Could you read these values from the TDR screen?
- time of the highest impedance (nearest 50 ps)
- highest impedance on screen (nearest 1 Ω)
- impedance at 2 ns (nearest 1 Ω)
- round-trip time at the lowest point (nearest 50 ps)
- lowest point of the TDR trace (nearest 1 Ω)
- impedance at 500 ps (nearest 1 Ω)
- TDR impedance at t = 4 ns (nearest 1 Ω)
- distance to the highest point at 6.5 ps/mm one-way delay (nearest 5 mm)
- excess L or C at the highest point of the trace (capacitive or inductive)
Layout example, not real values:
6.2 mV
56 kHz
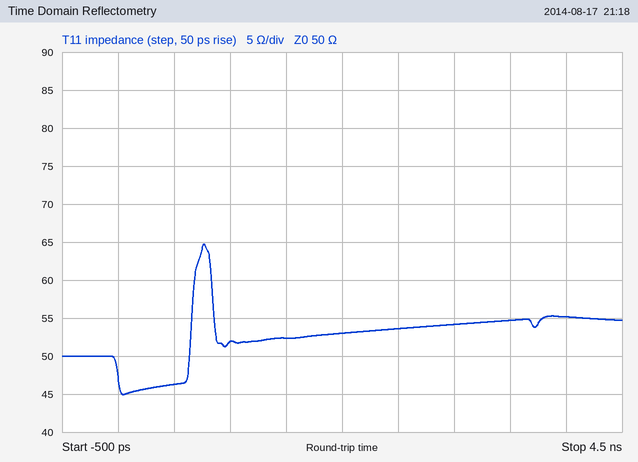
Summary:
750 ps
65 Ω
53 Ω
50 ps
45 Ω
46 Ω
55 Ω
60 mm
inductive
